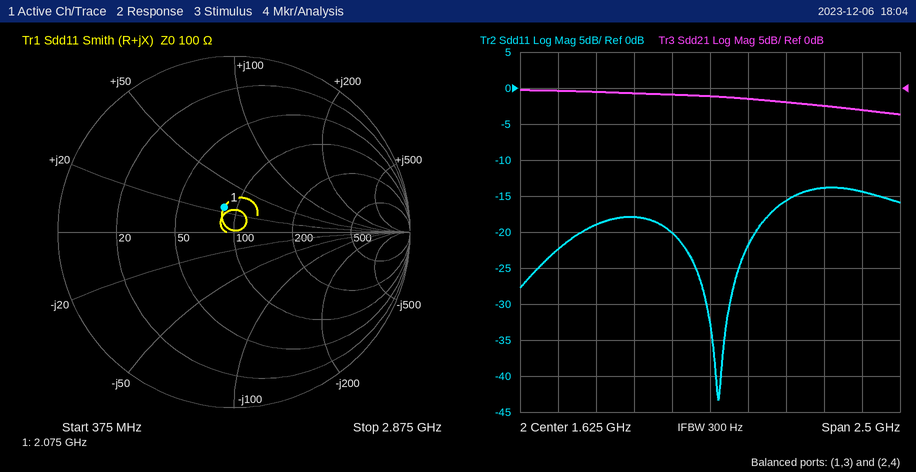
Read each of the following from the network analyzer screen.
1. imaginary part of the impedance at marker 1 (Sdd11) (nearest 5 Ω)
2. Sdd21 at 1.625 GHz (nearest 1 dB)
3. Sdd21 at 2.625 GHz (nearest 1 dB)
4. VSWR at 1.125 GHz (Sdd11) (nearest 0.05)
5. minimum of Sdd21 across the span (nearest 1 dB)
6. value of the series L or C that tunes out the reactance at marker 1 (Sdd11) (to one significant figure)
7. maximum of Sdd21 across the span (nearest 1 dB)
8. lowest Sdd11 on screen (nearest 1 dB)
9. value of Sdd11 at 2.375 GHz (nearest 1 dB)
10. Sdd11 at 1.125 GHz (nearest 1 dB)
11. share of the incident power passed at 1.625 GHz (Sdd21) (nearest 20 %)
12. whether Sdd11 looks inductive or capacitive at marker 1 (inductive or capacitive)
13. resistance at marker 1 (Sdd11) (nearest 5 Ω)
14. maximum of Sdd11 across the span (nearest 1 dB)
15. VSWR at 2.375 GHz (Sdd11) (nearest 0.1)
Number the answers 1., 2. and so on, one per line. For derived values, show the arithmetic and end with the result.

1. +25 Ω
2. -1 dB
3. -3 dB
4. |Γ| = 10^(-18/20) = 0.1259; VSWR = (1 + 0.1259)/(1 − 0.1259) ≈ 1.29, so 1.30 to the nearest 0.05
5. -4 dB
6. C = 1/(2π × 2.075 GHz × 25 Ω) ≈ 3 pF
7. 0 dB
8. -43 dB
9. -14 dB
10. -18 dB
11. 10^(-1/10) ≈ 79.4 %, so 80 % to the nearest 20 %
12. inductive
13. 85 Ω
14. -14 dB
15. |Γ| = 10^(-14/20) = 0.1995; VSWR = (1 + 0.1995)/(1 − 0.1995) ≈ 1.5
